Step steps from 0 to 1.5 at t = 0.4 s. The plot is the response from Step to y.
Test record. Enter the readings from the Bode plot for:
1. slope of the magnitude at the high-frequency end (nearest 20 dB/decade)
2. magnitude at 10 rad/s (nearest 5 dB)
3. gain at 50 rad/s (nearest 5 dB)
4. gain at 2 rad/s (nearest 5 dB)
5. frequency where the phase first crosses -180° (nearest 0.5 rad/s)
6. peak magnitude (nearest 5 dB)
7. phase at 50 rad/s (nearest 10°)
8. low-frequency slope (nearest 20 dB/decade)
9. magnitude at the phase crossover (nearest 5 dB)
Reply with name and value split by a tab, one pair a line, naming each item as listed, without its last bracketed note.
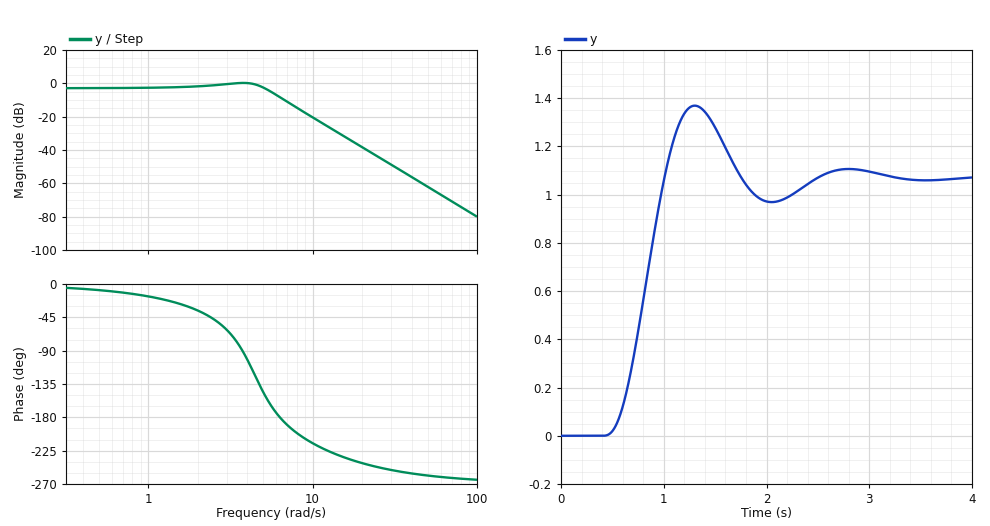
slope of the magnitude at the high-frequency end	-60 dB/decade
magnitude at 10 rad/s	-20 dB
gain at 50 rad/s	-60 dB
gain at 2 rad/s	0 dB
frequency where the phase first crosses -180°	6.5 rad/s
peak magnitude	0 dB
phase at 50 rad/s	-260°
low-frequency slope	0 dB/decade
magnitude at the phase crossover	-10 dB
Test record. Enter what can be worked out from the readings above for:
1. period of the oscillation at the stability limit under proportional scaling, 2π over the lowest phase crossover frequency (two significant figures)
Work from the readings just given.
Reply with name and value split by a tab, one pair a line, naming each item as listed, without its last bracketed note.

period of the oscillation at the stability limit under proportional scaling, 2π over the lowest phase crossover frequency	0.97 s
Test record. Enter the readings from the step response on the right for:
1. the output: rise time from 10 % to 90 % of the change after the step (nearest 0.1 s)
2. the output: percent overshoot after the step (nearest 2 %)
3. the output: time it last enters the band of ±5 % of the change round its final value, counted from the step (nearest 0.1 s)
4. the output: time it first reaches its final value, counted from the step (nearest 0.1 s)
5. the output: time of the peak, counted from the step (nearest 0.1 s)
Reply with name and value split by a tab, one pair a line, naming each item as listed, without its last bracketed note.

the output: rise time from 10 % to 90 % of the change after the step	0.4 s
the output: percent overshoot after the step	28 %
the output: time it last enters the band of ±5 % of the change round its final value, counted from the step	1.9 s
the output: time it first reaches its final value, counted from the step	0.6 s
the output: time of the peak, counted from the step	0.9 s
